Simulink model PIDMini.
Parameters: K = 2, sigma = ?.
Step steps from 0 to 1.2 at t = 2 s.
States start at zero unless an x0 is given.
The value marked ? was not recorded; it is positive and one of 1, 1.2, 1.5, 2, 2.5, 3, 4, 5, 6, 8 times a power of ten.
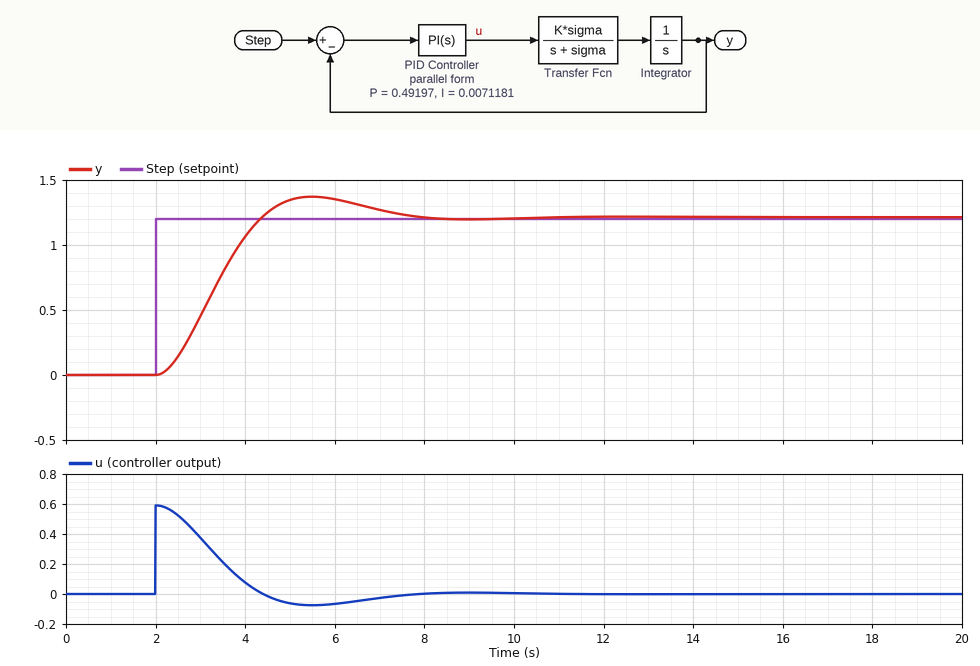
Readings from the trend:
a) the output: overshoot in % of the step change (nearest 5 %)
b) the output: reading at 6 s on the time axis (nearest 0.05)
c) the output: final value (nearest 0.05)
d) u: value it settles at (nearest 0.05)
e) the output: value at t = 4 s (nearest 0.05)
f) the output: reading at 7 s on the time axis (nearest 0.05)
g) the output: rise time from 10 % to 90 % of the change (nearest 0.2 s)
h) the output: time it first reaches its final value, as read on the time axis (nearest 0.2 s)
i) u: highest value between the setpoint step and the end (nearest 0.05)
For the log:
15 %
1.35
1.20
0.00
1.05
1.25
1.6 s
4.4 s
0.60
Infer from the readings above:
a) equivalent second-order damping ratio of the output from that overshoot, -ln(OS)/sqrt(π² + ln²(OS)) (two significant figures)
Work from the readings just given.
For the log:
0.52
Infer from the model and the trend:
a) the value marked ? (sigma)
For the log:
1.2
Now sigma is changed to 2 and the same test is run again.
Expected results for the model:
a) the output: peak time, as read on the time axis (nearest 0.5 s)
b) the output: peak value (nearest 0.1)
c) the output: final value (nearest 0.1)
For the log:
5.0 s
1.3
1.2
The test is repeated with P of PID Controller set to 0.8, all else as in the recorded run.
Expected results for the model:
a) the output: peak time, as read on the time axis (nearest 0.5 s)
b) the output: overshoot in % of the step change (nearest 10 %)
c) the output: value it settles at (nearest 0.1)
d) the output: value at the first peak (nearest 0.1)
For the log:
4.5 s
20 %
1.2
1.5
